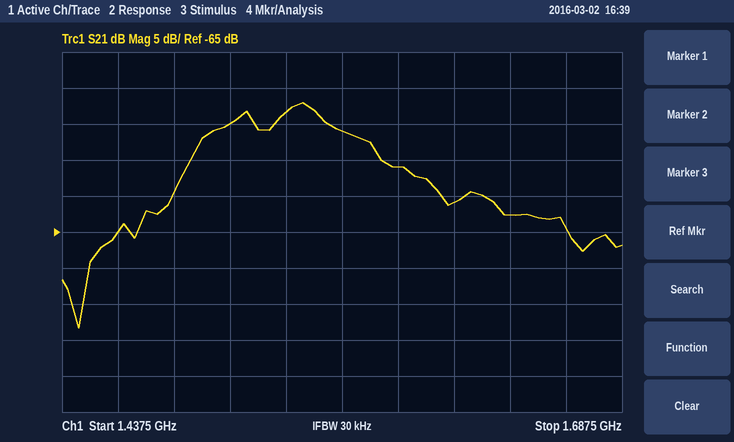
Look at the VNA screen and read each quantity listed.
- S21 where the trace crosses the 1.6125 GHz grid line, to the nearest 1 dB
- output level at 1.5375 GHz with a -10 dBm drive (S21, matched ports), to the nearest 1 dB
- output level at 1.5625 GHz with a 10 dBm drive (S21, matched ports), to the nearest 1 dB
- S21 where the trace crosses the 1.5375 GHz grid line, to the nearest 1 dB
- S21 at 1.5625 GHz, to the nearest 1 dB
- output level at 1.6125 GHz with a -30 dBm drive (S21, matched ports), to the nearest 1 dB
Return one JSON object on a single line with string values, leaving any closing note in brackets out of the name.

{"S21 where the trace crosses the 1.6125 GHz grid line, to the nearest 1 dB": "-61 dB", "output level at 1.5375 GHz with a -10 dBm drive (S21, matched ports), to the nearest 1 dB": "-58 dBm", "output level at 1.5625 GHz with a 10 dBm drive (S21, matched ports), to the nearest 1 dB": "-41 dBm", "S21 where the trace crosses the 1.5375 GHz grid line, to the nearest 1 dB": "-48 dB", "S21 at 1.5625 GHz, to the nearest 1 dB": "-51 dB", "output level at 1.6125 GHz with a -30 dBm drive (S21, matched ports), to the nearest 1 dB": "-91 dBm"}
